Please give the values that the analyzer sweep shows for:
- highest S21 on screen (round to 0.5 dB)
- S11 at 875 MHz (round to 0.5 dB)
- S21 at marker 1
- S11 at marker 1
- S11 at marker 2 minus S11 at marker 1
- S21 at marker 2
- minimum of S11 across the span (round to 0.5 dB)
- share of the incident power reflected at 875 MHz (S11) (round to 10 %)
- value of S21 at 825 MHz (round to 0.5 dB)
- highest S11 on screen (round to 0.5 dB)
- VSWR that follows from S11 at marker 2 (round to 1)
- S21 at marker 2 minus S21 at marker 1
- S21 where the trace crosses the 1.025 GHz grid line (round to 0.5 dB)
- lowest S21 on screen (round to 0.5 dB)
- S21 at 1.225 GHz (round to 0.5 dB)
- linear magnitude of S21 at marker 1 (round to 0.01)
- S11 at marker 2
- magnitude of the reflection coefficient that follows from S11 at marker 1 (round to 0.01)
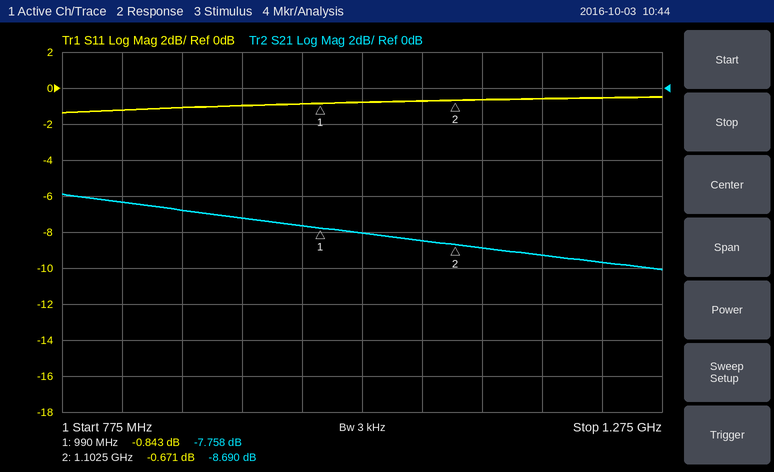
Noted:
-6.0 dB
-1.0 dB
-7.758 dB
-0.843 dB
0.172 dB
-8.690 dB
-1.5 dB
80 %
-6.5 dB
-0.5 dB
26
-0.932 dB
-8.0 dB
-10.0 dB
-9.5 dB
0.41
-0.671 dB
0.91
